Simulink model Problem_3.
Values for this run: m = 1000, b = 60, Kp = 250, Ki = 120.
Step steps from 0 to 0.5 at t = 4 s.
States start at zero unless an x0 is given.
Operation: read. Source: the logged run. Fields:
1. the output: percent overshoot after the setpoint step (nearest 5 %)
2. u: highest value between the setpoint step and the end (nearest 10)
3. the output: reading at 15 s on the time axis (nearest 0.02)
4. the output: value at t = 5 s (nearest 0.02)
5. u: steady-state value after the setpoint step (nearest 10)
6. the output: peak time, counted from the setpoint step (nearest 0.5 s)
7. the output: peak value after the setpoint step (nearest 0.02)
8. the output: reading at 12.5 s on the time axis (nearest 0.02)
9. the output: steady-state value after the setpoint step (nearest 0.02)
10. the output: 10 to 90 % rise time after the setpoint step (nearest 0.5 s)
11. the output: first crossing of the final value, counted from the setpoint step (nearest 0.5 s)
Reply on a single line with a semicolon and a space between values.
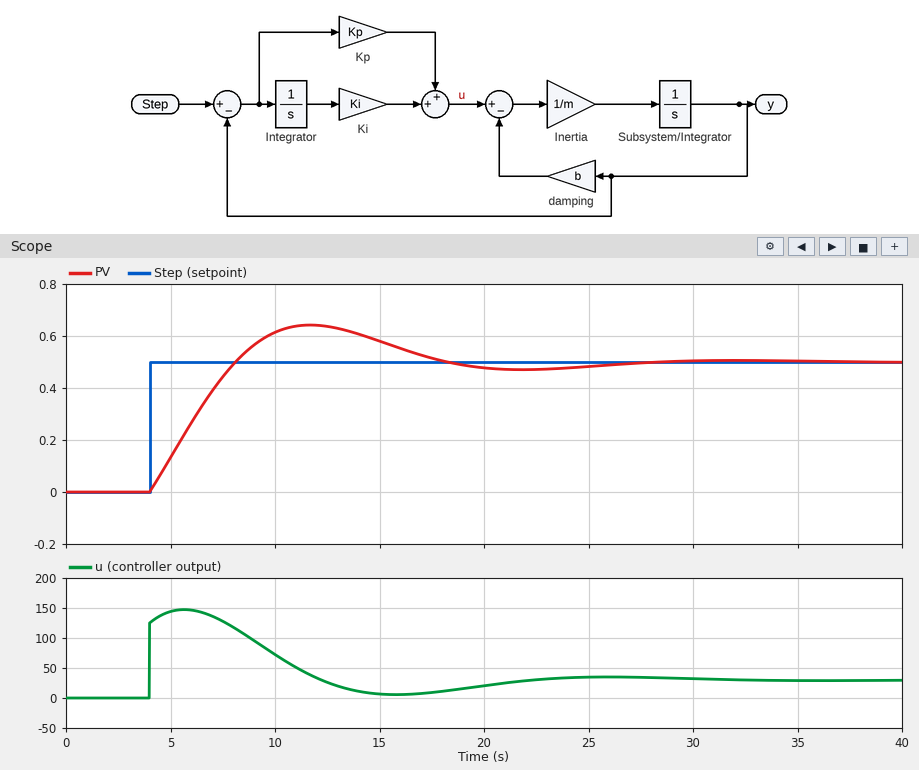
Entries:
30 %; 150; 0.58; 0.14; 30; 7.5 s; 0.64; 0.64; 0.50; 3.0 s; 4.0 s
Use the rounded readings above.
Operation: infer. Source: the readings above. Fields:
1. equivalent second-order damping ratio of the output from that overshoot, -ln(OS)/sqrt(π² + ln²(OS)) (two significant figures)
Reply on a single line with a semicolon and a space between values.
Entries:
0.36
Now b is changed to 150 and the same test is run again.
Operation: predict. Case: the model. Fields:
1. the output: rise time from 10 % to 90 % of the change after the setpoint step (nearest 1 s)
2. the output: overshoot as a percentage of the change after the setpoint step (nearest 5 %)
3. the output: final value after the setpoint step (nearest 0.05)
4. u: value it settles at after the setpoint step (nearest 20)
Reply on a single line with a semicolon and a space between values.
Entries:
4 s; 15 %; 0.50; 80
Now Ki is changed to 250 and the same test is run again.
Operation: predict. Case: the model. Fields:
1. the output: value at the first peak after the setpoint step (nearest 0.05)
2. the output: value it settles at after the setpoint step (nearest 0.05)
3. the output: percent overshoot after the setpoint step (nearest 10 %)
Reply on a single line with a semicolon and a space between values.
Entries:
0.70; 0.50; 40 %
